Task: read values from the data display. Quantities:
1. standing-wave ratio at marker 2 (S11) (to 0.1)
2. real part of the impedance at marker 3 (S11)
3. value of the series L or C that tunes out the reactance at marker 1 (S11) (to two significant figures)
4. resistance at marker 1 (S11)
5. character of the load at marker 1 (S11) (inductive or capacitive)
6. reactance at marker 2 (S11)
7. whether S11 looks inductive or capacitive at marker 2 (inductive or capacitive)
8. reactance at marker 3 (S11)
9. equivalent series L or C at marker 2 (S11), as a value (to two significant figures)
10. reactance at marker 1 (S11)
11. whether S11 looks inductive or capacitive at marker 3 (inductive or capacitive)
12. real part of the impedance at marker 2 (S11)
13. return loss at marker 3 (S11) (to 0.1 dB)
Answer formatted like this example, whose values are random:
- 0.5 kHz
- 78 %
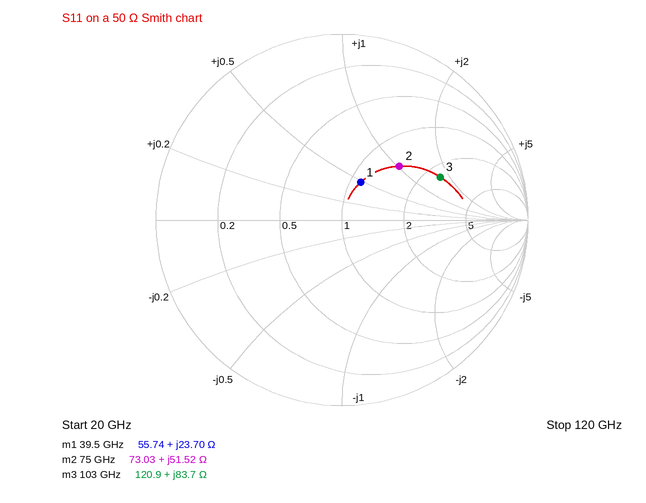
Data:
- 2.5
- 120.9 Ω
- 170 fF
- 55.74 Ω
- inductive
- +51.52 Ω
- inductive
- +83.7 Ω
- 110 pH
- +23.70 Ω
- inductive
- 73.03 Ω
- 4.8 dB
